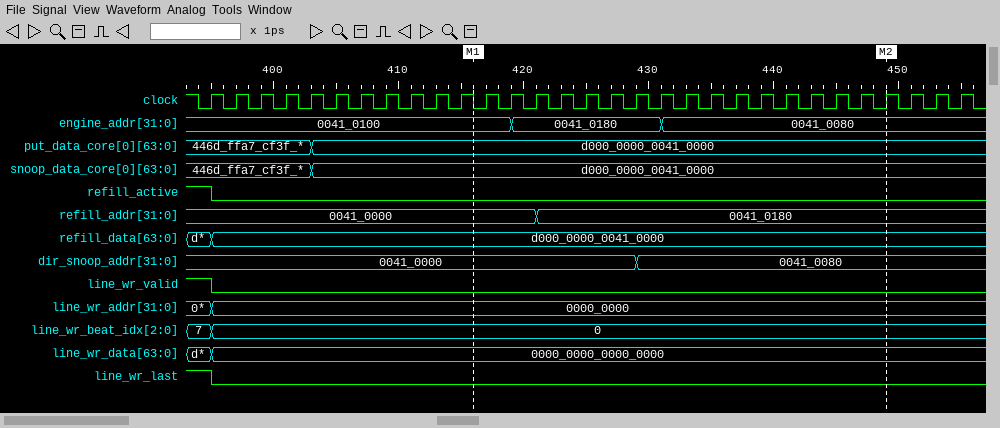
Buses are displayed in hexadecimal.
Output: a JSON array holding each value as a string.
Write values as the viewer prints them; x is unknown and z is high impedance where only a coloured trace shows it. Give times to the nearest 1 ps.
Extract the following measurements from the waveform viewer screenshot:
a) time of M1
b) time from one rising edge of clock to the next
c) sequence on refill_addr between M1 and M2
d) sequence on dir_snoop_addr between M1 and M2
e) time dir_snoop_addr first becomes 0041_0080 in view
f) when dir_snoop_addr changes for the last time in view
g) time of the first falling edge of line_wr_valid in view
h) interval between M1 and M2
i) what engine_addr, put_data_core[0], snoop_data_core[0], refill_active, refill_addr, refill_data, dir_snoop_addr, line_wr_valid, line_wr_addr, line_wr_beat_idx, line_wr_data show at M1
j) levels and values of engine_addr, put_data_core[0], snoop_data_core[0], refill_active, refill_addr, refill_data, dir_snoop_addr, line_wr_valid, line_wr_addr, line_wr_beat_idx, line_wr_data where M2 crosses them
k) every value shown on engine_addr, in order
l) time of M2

["416 ps", "2 ps", "0041_0000, 0041_0180", "0041_0000, 0041_0080", "429 ps", "429 ps", "395 ps", "33 ps", "engine_addr=0041_0100, put_data_core[0]=d000_0000_0041_0000, snoop_data_core[0]=d000_0000_0041_0000, refill_active=0, refill_addr=0041_0000, refill_data=d000_0000_0041_0000, dir_snoop_addr=0041_0000, line_wr_valid=0, line_wr_addr=0000_0000, line_wr_beat_idx=0, line_wr_data=0000_0000_0000_0000", "engine_addr=0041_0080, put_data_core[0]=d000_0000_0041_0000, snoop_data_core[0]=d000_0000_0041_0000, refill_active=0, refill_addr=0041_0180, refill_data=d000_0000_0041_0000, dir_snoop_addr=0041_0080, line_wr_valid=0, line_wr_addr=0000_0000, line_wr_beat_idx=0, line_wr_data=0000_0000_0000_0000", "0041_0100, 0041_0180, 0041_0080", "449 ps"]
